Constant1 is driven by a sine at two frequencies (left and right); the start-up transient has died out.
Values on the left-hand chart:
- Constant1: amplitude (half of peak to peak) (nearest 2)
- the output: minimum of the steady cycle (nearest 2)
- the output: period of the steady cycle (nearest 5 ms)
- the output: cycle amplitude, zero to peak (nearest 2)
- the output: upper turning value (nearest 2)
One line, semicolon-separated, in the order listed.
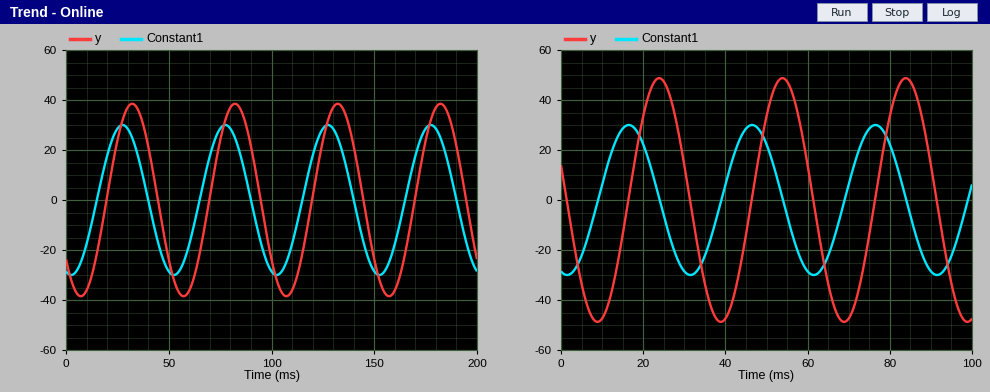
30; -38; 50 ms; 38; 38
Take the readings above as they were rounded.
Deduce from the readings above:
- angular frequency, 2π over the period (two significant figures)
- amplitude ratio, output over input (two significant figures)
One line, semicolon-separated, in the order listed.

0.13 rad/ms; 1.3
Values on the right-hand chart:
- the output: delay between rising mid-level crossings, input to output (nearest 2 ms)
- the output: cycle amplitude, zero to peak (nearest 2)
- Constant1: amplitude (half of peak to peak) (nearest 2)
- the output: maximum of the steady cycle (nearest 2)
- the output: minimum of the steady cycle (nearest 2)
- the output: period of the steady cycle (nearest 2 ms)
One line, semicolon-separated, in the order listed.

8 ms; 48; 30; 48; -48; 30 ms
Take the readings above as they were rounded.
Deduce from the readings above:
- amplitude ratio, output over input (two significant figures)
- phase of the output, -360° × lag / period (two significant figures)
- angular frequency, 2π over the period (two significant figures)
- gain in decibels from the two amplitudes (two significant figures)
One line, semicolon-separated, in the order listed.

1.6; -96°; 0.21 rad/ms; 4.1 dB
